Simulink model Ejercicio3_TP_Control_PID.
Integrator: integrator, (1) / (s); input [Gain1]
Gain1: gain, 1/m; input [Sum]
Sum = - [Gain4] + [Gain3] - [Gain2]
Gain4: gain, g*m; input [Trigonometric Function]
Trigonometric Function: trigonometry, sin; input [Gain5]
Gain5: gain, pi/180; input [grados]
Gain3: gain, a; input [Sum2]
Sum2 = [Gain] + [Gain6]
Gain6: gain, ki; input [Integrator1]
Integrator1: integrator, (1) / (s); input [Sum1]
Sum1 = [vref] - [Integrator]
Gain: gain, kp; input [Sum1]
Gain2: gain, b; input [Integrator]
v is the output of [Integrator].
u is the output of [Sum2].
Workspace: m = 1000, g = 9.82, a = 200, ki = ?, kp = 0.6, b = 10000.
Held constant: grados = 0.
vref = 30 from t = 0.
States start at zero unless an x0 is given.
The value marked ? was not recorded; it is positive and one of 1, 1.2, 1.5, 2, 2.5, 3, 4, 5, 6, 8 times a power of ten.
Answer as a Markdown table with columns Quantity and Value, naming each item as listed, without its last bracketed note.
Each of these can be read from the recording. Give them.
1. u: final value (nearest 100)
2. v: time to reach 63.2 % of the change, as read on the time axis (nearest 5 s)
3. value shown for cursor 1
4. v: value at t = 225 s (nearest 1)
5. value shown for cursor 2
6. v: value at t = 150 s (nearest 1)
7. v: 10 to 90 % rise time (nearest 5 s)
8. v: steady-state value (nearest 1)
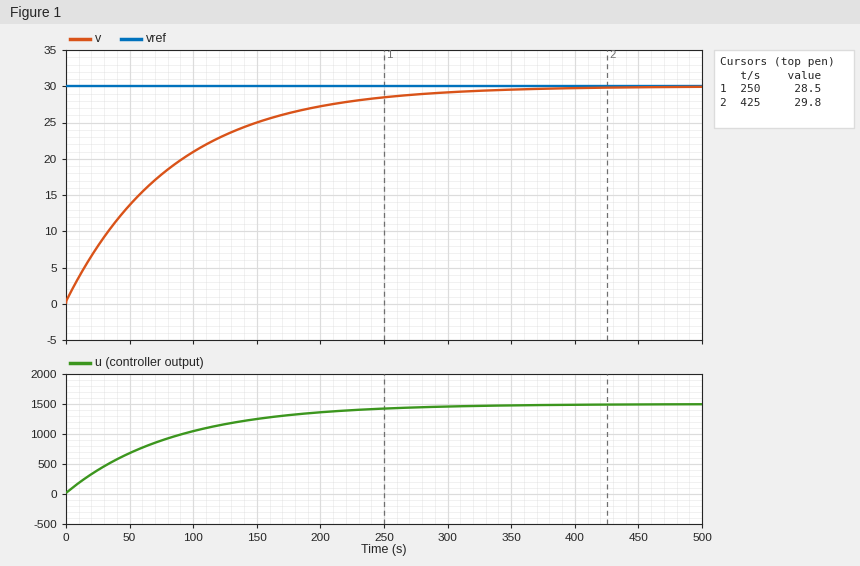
| Quantity | Value |
|---|---|
| u: final value | 1500 |
| v: time to reach 63.2 % of the change, as read on the time axis | 85 s |
| value shown for cursor 1 | 28.5 |
| v: value at t = 225 s | 28 |
| value shown for cursor 2 | 29.8 |
| v: value at t = 150 s | 25 |
| v: 10 to 90 % rise time | 185 s |
| v: steady-state value | 30 |
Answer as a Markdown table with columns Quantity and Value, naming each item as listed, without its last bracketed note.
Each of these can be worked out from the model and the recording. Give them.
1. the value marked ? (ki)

| Quantity | Value |
|---|---|
| the value marked ? | 0.6 |
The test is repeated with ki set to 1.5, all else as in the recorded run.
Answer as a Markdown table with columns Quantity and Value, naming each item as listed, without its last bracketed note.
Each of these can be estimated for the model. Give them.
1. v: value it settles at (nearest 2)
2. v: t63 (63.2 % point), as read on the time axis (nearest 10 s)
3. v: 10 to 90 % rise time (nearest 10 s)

| Quantity | Value |
|---|---|
| v: value it settles at | 30 |
| v: t63 (63.2 % point), as read on the time axis | 30 s |
| v: 10 to 90 % rise time | 70 s |
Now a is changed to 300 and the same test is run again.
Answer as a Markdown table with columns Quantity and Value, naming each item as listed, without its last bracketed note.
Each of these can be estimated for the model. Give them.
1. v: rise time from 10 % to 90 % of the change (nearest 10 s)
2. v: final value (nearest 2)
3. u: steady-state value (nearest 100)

| Quantity | Value |
|---|---|
| v: rise time from 10 % to 90 % of the change | 120 s |
| v: final value | 30 |
| u: steady-state value | 1000 |
